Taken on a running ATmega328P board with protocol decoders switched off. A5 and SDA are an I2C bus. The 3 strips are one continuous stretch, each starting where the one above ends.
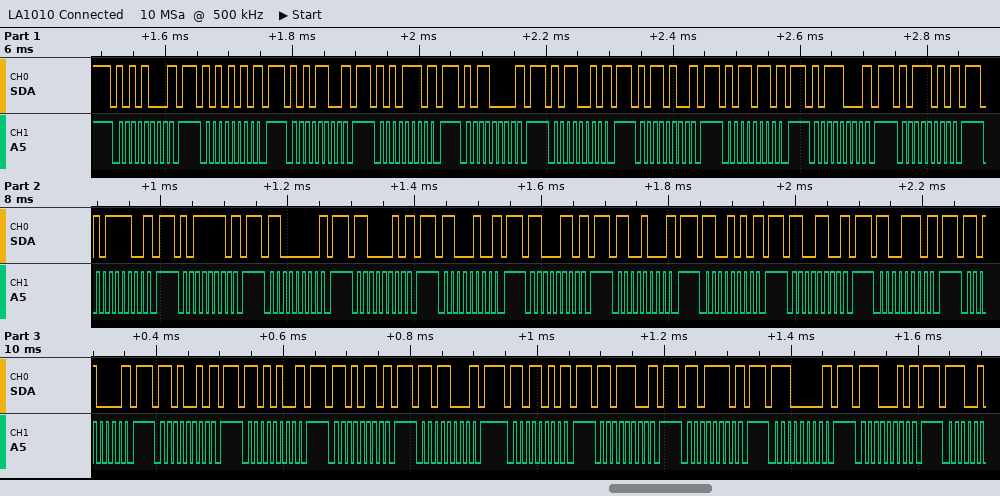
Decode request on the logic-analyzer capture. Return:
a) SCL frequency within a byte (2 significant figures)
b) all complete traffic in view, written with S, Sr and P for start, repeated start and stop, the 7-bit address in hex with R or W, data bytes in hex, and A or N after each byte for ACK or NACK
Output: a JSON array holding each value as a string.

["100 kHz", "S 54W N P S 55W N P S 56W N P S 57W N P S 58W N P S 59W N P S 5AW N P S 5BW N P S 5CW N P S 5DW N P S 5EW N P S 5FW N P S 60W N P S 61W N P S 62W N P S 63W N P S 64W N P S 65W N P S 66W N P S 67W N P S 68W N P S 69W N P S 6AW N P S 6BW N P S 6CW N P S 6DW N P S 6EW N P S 6FW N P S 70W N P S 71W N P"]
